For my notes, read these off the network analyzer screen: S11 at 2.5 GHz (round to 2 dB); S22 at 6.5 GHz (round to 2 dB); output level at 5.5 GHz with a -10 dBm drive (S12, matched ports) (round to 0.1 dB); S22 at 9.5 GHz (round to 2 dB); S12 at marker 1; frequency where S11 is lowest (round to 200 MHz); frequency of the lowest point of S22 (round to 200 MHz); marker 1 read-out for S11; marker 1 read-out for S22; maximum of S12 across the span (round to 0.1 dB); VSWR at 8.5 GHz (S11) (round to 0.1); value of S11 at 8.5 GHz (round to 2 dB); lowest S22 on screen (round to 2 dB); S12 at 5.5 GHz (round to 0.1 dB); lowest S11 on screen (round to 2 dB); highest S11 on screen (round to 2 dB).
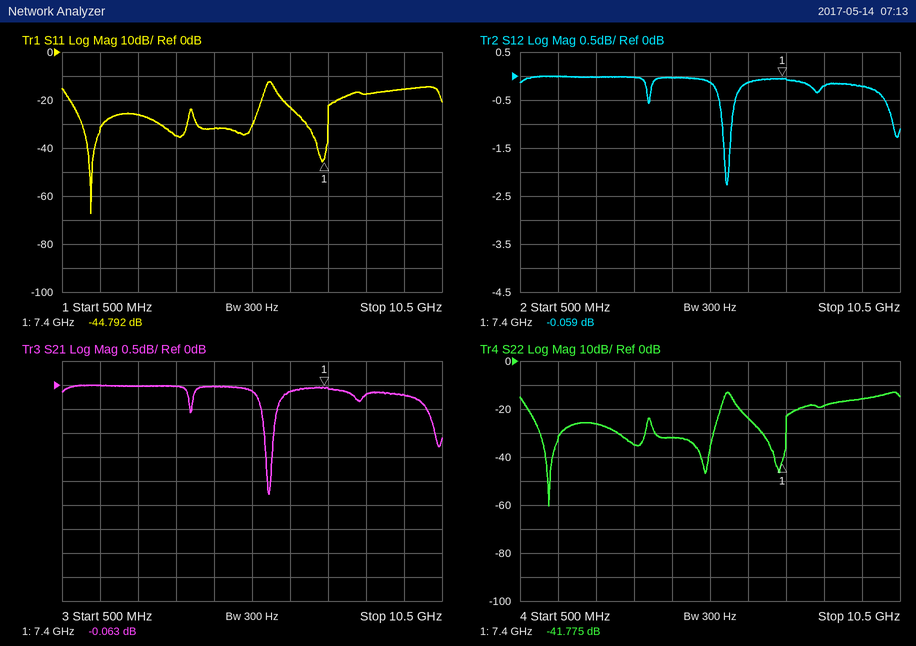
-26 dB
-24 dB
-10.1 dBm
-16 dB
-0.059 dB
1.2 GHz
1.2 GHz
-44.792 dB
-41.775 dB
0.0 dB
1.3
-18 dB
-60 dB
-0.1 dB
-68 dB
-12 dB
